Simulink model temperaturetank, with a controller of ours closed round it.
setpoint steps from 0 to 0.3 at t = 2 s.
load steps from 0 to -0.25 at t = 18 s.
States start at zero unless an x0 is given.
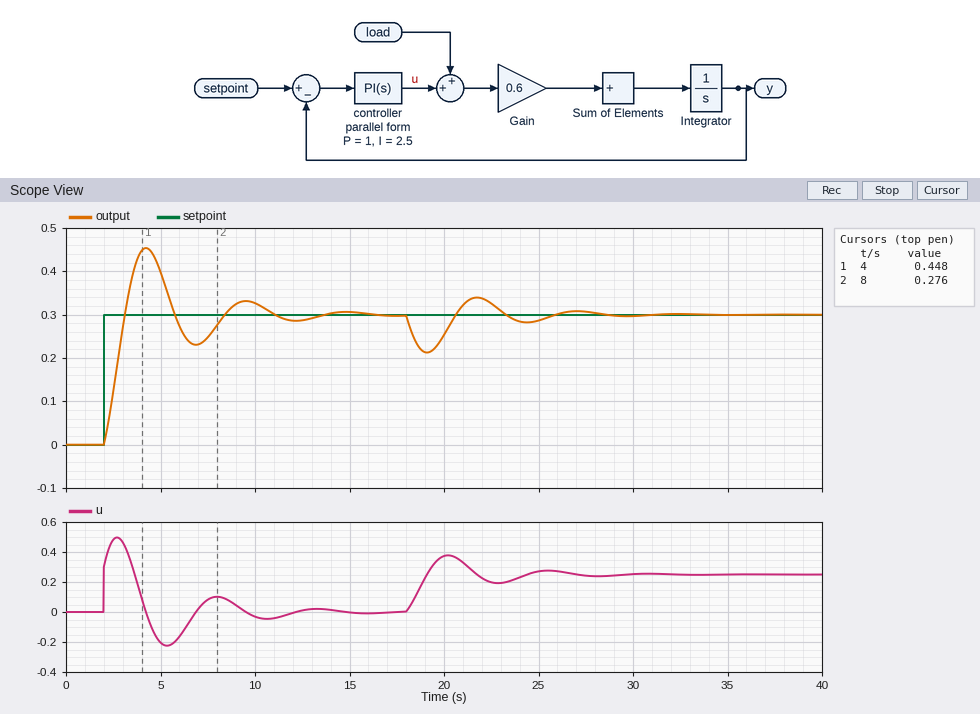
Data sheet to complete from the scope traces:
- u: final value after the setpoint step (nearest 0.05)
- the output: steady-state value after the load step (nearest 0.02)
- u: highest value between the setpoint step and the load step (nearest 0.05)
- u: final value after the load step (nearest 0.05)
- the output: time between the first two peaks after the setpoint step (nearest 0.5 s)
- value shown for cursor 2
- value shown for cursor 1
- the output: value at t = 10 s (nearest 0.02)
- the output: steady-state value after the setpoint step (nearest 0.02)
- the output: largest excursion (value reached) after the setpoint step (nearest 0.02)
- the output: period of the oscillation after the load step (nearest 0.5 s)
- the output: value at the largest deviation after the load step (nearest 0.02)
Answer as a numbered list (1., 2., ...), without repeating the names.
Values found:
1. 0.00
2. 0.30
3. 0.50
4. 0.25
5. 5.5 s
6. 0.276
7. 0.448
8. 0.32
9. 0.30
10. 0.46
11. 5.5 s
12. 0.22
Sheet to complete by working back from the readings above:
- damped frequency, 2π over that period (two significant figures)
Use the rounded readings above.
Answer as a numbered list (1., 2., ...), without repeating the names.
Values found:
1. 1.1 rad/s
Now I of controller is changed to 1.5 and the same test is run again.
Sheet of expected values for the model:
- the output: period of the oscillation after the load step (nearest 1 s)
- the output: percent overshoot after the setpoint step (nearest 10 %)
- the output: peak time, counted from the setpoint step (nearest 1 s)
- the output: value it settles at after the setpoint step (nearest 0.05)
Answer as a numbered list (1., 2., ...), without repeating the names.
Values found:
1. 7 s
2. 40 %
3. 3 s
4. 0.30
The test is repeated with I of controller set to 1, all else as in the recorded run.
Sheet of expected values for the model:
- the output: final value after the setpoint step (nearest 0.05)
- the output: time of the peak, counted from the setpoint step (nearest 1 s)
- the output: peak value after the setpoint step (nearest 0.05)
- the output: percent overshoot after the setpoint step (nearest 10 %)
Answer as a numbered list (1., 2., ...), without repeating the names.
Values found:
1. 0.30
2. 3 s
3. 0.40
4. 40 %
